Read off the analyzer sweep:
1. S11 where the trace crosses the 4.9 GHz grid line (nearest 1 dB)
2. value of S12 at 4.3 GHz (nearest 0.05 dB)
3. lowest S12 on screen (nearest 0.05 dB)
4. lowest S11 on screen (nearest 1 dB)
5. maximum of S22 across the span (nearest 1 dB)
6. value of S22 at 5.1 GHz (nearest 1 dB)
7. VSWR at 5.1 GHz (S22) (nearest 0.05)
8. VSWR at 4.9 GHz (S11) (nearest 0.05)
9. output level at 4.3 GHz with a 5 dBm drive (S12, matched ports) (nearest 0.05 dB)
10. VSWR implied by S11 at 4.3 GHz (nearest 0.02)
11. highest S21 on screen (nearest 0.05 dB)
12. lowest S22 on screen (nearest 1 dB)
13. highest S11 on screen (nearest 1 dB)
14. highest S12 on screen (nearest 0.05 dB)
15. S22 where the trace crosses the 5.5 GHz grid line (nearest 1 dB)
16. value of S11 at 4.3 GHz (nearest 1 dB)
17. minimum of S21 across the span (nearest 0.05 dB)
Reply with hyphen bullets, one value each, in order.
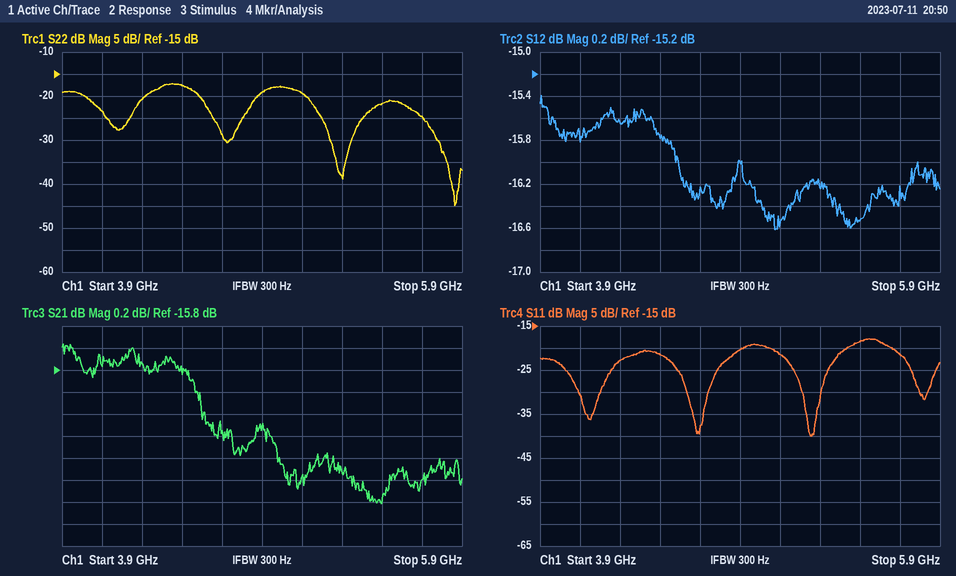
- -20 dB
- -15.65 dB
- -16.60 dB
- -40 dB
- -17 dB
- -19 dB
- 1.25
- 1.20
- -10.65 dBm
- 1.16
- -15.55 dB
- -45 dB
- -18 dB
- -15.40 dB
- -22 dB
- -23 dB
- -17.00 dB
